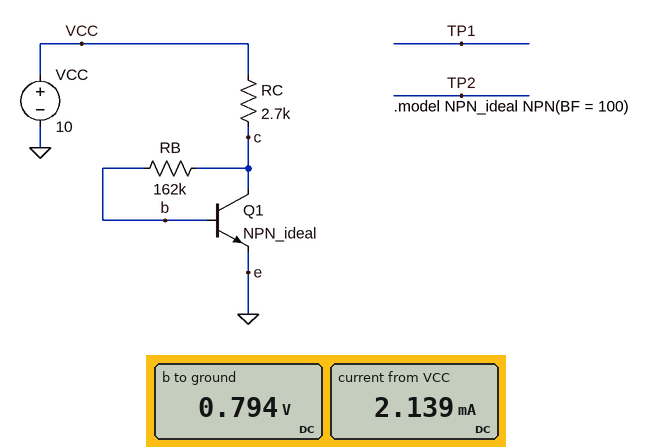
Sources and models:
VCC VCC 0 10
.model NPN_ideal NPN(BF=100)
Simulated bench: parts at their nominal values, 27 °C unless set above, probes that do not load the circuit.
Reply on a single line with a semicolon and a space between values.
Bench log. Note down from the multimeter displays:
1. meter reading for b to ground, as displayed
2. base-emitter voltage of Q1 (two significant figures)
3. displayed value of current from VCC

0.794 V; 790 mV; 2.139 mA
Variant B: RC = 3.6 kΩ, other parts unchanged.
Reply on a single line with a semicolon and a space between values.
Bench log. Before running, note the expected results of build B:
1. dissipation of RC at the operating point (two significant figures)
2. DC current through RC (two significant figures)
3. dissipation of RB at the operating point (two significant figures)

11 mW; 1.8 mA; 50 µW
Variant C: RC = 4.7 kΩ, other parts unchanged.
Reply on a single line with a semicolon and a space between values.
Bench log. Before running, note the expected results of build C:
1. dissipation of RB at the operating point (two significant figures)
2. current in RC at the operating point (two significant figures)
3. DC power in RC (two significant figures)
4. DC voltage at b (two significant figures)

34 µW; 1.5 mA; 10 mW; 780 mV
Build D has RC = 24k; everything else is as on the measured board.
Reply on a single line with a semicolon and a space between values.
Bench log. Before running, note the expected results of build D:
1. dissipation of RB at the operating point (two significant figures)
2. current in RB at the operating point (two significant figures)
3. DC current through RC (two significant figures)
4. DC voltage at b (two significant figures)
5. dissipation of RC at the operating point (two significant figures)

2.1 µW; 3.6 µA; 360 µA; 750 mV; 3.1 mW
